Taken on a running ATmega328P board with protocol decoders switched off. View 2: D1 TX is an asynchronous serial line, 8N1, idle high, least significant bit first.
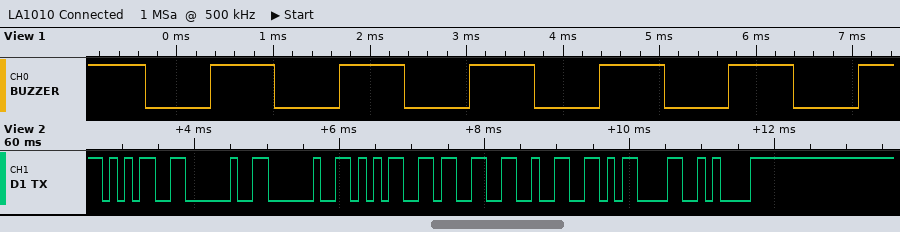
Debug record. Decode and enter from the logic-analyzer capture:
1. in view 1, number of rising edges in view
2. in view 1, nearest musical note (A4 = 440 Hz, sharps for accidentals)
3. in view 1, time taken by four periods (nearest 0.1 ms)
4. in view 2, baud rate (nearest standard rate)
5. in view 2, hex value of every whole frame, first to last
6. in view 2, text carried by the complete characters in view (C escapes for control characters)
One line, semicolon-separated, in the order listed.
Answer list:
6; F#5; 5.4 ms; 9600 baud; 35 20 20 35 33 32 0D 0A; "5  532\r\n"
